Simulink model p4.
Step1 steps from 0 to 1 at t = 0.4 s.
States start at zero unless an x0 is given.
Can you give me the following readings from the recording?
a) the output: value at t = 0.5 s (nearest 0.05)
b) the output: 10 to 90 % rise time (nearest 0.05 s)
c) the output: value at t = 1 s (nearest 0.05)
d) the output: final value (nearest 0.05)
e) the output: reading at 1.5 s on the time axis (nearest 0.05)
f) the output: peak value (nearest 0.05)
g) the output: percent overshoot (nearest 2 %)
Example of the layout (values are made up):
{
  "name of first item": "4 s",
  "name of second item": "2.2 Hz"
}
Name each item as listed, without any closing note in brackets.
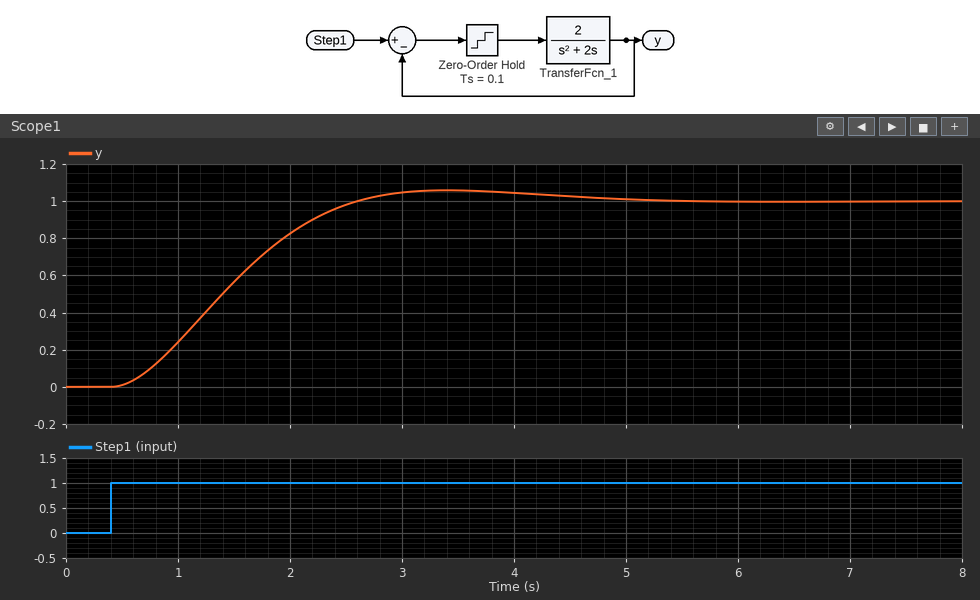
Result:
{
  "the output: value at t = 0.5 s": "0.00",
  "the output: 10 to 90 % rise time": "1.45 s",
  "the output: value at t = 1 s": "0.25",
  "the output: final value": "1.00",
  "the output: reading at 1.5 s on the time axis": "0.55",
  "the output: peak value": "1.05",
  "the output: percent overshoot": "6 %"
}
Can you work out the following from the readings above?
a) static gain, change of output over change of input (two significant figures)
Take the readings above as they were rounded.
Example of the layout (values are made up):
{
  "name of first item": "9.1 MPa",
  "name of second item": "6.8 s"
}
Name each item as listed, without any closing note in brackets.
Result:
{
  "static gain, change of output over change of input": "1.0"
}
